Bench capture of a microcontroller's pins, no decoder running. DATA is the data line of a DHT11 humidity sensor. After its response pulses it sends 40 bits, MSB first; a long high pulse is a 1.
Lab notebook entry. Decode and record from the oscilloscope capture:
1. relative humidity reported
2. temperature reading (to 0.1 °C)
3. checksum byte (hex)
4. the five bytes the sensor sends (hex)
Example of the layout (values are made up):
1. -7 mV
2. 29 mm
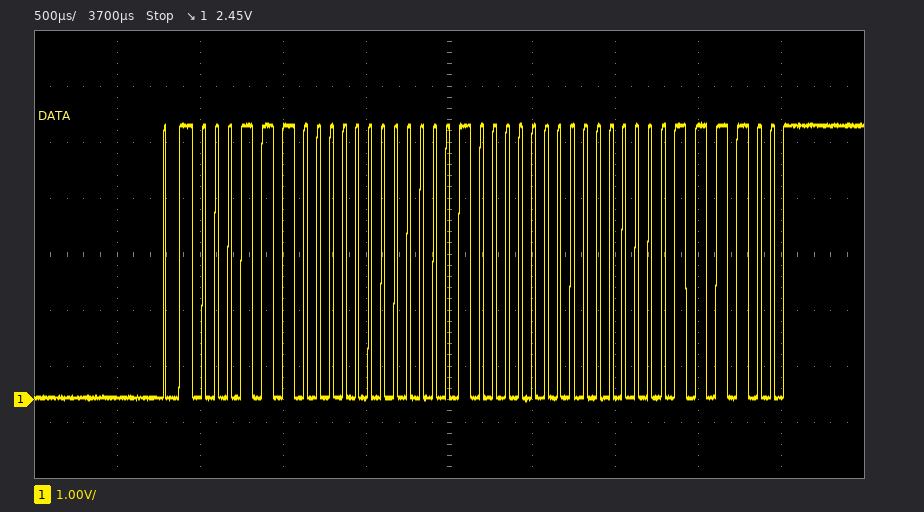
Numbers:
1. 28 %
2. 32.0 °C
3. 0x3C
4. 1C 00 20 00 3C
